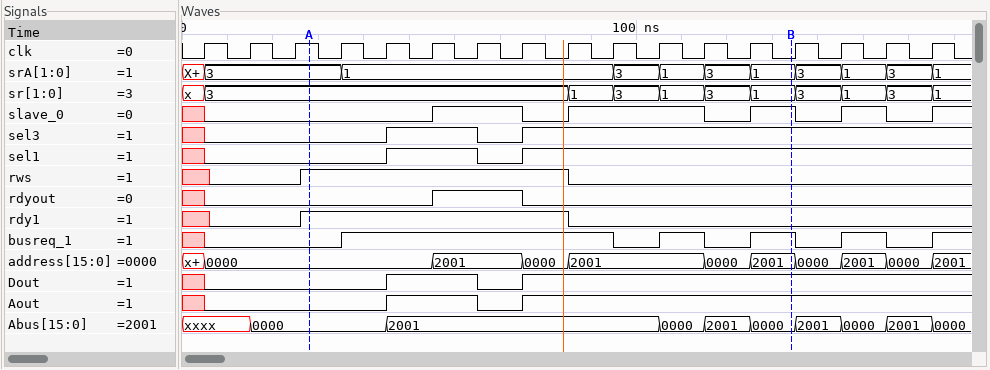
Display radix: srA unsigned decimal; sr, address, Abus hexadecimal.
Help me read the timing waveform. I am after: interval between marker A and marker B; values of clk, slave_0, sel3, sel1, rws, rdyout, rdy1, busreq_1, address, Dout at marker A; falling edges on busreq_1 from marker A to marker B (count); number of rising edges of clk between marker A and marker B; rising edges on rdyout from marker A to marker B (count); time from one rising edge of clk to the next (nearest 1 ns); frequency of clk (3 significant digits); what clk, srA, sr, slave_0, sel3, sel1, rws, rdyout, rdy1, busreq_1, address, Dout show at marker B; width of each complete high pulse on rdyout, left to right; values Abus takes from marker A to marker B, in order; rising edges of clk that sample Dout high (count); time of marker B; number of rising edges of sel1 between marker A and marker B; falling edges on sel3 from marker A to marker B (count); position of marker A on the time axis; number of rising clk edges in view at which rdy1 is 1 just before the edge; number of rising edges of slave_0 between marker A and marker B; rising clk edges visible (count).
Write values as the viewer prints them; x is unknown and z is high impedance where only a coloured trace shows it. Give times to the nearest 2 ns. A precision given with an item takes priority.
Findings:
106 ns
clk=1, slave_0=0, sel3=0, sel1=0, rws=1, rdyout=0, rdy1=1, busreq_1=0, address=0000, Dout=0
2
10
1
10 ns
100 MHz
clk=0, srA=1, sr=1, slave_0=1, sel3=1, sel1=1, rws=0, rdyout=0, rdy1=0, busreq_1=1, address=2001, Dout=1
20 ns
0000, 2001, 0000, 2001, 0000
11
134 ns
2
1
28 ns
6
3
17
